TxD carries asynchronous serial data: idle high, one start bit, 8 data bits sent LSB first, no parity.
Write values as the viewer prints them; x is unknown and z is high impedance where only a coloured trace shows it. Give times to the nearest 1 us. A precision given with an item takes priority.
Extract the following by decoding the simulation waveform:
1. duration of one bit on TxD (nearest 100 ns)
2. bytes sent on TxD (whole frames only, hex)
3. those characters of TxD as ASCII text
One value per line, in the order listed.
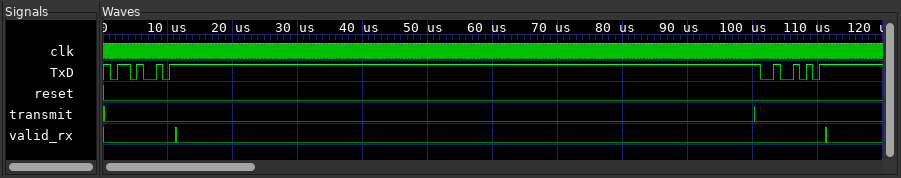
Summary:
1000 ns
4B, 52
"KR"
